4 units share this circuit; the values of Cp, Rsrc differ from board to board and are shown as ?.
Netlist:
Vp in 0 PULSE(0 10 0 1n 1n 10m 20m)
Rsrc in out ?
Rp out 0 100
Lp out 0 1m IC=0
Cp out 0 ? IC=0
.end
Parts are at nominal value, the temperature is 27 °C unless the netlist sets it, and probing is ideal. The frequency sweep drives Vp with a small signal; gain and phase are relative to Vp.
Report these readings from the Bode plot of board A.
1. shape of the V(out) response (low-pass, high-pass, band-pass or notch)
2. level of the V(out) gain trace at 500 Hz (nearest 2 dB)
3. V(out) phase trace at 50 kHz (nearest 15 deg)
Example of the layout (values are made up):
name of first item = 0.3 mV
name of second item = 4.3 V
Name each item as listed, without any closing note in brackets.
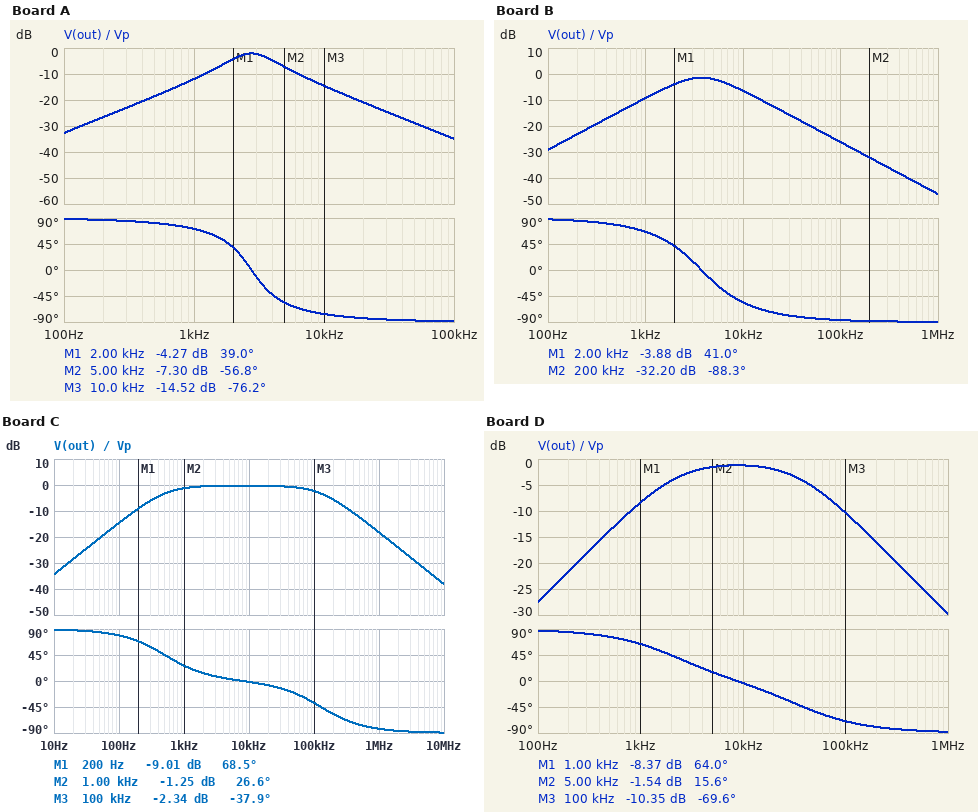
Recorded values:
shape of the V(out) response = band-pass
level of the V(out) gain trace at 500 Hz = -18 dB
V(out) phase trace at 50 kHz = -90 deg
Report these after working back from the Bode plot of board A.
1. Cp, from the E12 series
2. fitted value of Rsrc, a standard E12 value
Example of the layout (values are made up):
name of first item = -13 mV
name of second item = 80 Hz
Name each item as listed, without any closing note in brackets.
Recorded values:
Cp, from the E12 series = 3.3 µF
fitted value of Rsrc, a standard E12 value = 27 Ω
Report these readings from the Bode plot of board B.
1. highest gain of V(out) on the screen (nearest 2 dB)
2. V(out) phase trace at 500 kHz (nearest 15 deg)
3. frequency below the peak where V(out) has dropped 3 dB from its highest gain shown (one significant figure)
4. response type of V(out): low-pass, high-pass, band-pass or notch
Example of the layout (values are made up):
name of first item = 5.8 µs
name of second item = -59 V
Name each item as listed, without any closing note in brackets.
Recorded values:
highest gain of V(out) on the screen = -2 dB
V(out) phase trace at 500 kHz = -90 deg
frequency below the peak where V(out) has dropped 3 dB from its highest gain shown = 2 kHz
response type of V(out): low-pass, high-pass, band-pass or notch = band-pass
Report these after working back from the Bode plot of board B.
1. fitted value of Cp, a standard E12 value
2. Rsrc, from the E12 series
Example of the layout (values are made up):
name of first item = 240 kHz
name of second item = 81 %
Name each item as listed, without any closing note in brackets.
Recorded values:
fitted value of Cp, a standard E12 value = 1.8 µF
Rsrc, from the E12 series = 18 Ω
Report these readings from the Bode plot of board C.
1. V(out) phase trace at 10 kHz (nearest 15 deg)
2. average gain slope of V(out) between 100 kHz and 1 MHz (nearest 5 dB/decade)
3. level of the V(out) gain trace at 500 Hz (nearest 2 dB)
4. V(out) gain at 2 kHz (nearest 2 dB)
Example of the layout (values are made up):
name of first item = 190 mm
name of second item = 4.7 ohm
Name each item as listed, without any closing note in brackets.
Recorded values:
V(out) phase trace at 10 kHz = 0 deg
average gain slope of V(out) between 100 kHz and 1 MHz = -15 dB/decade
level of the V(out) gain trace at 500 Hz = -4 dB
V(out) gain at 2 kHz = 0 dB
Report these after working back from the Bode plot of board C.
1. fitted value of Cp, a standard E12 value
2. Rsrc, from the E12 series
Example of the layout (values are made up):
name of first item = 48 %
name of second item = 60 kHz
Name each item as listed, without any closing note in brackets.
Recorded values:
fitted value of Cp, a standard E12 value = 390 nF
Rsrc, from the E12 series = 3.3 Ω
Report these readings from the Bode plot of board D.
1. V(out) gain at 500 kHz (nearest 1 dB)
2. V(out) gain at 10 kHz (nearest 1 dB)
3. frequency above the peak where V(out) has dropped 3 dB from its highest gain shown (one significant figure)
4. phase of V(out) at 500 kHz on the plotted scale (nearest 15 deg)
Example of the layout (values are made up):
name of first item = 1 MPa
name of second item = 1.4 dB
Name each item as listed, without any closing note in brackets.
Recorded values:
V(out) gain at 500 kHz = -24 dB
V(out) gain at 10 kHz = -1 dB
frequency above the peak where V(out) has dropped 3 dB from its highest gain shown = 40 kHz
phase of V(out) at 500 kHz on the plotted scale = -90 deg
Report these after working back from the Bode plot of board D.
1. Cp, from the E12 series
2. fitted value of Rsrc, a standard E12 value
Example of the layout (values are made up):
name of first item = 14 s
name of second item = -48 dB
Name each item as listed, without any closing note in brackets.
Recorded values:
Cp, from the E12 series = 330 nF
fitted value of Rsrc, a standard E12 value = 15 Ω
